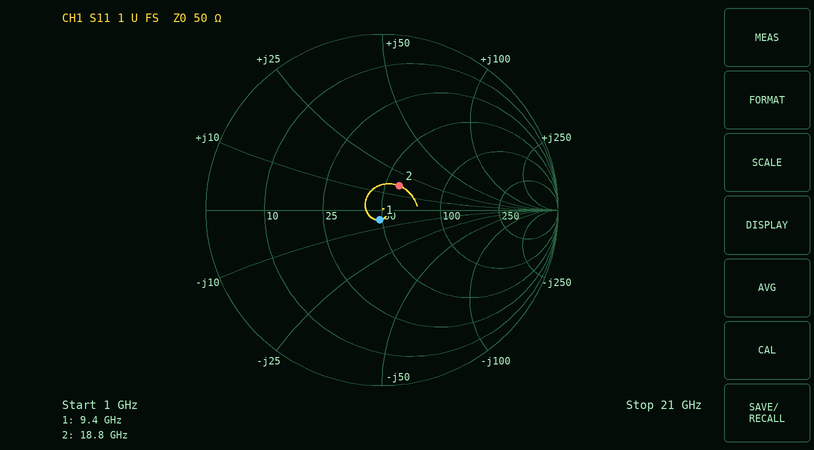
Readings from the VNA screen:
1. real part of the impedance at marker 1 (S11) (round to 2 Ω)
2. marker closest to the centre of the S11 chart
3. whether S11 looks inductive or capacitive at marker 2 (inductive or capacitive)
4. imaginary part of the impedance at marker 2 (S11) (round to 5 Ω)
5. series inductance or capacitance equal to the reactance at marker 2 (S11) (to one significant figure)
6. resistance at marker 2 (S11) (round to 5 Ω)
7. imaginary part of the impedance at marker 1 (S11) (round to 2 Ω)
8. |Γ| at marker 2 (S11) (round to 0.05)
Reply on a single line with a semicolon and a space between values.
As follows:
48 Ω; marker 1; inductive; +15 Ω; 100 pH; 60 Ω; -6 Ω; 0.15
